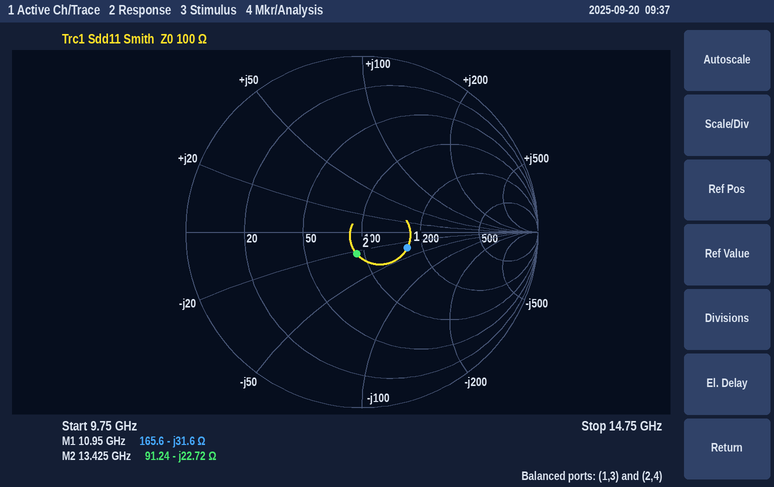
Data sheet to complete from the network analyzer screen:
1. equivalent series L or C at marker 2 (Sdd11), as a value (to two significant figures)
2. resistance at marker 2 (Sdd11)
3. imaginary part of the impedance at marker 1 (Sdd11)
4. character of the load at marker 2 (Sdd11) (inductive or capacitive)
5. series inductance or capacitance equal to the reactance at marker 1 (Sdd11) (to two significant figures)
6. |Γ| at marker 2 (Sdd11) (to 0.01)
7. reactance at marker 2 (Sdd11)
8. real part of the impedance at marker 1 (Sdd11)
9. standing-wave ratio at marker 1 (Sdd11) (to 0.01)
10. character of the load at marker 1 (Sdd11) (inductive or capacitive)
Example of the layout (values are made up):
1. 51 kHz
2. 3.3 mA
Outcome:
1. 520 fF
2. 91.24 Ω
3. -31.6 Ω
4. capacitive
5. 460 fF
6. 0.13
7. -22.72 Ω
8. 165.6 Ω
9. 1.75
10. capacitive
